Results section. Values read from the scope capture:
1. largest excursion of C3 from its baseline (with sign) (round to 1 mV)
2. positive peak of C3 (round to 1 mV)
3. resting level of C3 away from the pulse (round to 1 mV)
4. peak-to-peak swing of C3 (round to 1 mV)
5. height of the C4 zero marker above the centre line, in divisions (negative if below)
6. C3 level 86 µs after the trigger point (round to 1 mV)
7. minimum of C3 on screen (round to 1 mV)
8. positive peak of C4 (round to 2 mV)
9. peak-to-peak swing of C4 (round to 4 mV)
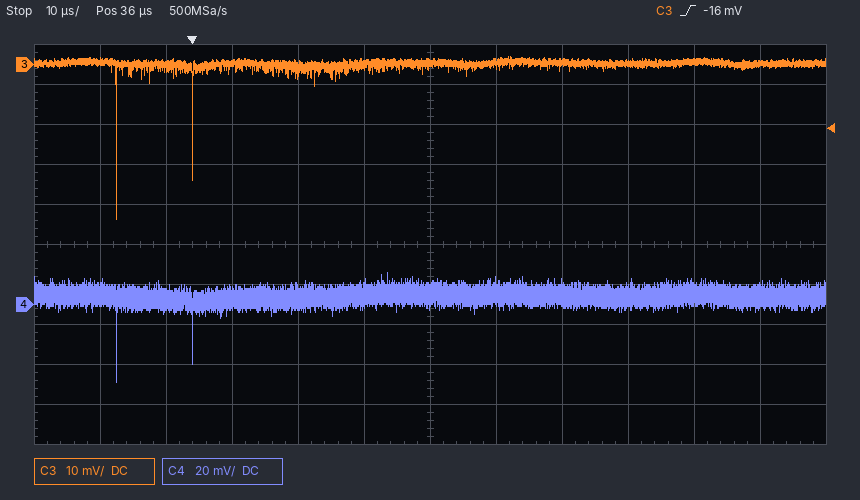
-39 mV
2 mV
0 mV
41 mV
-1.5 div
0 mV
-39 mV
16 mV
56 mV
